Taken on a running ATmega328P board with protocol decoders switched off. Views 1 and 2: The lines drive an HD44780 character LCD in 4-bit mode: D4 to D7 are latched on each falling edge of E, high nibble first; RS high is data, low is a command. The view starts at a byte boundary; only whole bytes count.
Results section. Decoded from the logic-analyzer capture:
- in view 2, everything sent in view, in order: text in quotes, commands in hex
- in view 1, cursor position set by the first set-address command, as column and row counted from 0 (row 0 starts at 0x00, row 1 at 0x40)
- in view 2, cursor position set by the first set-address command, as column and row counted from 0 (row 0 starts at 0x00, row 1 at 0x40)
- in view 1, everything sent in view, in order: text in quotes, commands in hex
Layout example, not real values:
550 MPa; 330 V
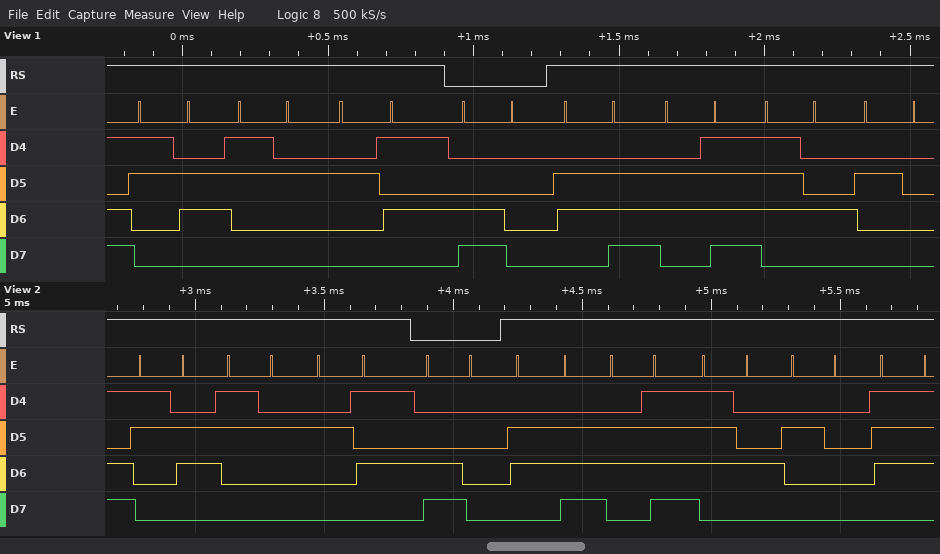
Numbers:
"62%" 0xC0 "not w"; column 0, row 1; column 0, row 1; "62%" 0xC0 "not "
